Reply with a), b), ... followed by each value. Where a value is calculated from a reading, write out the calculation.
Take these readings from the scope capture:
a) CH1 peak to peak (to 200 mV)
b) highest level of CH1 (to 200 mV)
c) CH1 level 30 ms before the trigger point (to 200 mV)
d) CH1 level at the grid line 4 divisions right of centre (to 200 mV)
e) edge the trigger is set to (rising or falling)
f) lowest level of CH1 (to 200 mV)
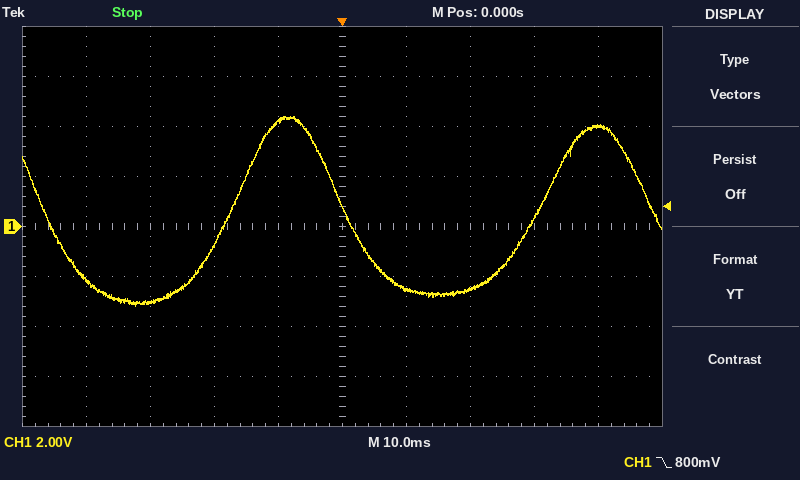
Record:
a) 4.4 V − (-3.2 V) = 7.6 V
b) 4.4 V
c) -3.0 V
d) 4.0 V
e) falling
f) -3.2 V
